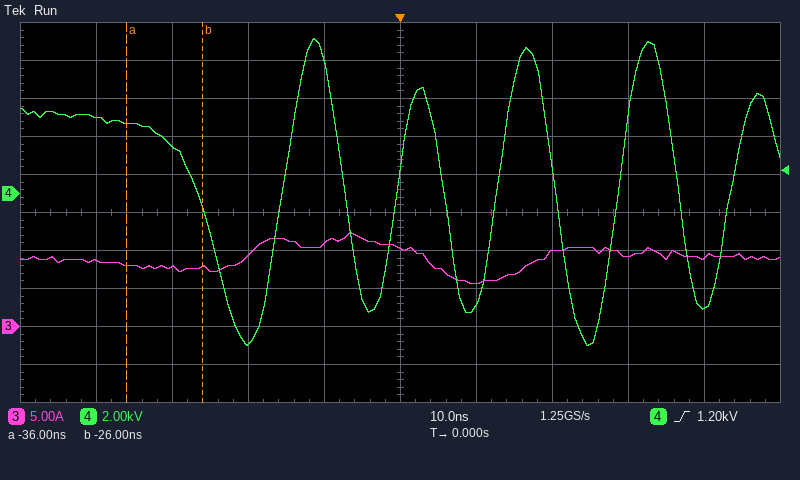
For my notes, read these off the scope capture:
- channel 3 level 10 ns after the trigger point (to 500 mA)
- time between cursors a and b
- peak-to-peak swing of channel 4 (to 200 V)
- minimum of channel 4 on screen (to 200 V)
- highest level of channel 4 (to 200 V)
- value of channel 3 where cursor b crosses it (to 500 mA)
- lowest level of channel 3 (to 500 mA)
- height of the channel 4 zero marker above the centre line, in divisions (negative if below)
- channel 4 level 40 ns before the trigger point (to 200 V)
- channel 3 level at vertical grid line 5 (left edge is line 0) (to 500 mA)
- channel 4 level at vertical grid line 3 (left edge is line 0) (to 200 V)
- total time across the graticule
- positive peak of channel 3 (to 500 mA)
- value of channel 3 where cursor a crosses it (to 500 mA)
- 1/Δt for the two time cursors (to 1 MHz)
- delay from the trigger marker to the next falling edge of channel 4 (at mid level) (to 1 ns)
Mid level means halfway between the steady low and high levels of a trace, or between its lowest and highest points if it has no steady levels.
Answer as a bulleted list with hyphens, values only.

- 5.5 A
- 10 ns
- 16.2 kV
- -8.0 kV
- 8.2 kV
- 8.0 A
- 5.5 A
- +0.5 div
- 4.0 kV
- 10.5 A
- -7.8 kV
- 100 ns
- 12.5 A
- 8.0 A
- 100 MHz
- 6 ns
